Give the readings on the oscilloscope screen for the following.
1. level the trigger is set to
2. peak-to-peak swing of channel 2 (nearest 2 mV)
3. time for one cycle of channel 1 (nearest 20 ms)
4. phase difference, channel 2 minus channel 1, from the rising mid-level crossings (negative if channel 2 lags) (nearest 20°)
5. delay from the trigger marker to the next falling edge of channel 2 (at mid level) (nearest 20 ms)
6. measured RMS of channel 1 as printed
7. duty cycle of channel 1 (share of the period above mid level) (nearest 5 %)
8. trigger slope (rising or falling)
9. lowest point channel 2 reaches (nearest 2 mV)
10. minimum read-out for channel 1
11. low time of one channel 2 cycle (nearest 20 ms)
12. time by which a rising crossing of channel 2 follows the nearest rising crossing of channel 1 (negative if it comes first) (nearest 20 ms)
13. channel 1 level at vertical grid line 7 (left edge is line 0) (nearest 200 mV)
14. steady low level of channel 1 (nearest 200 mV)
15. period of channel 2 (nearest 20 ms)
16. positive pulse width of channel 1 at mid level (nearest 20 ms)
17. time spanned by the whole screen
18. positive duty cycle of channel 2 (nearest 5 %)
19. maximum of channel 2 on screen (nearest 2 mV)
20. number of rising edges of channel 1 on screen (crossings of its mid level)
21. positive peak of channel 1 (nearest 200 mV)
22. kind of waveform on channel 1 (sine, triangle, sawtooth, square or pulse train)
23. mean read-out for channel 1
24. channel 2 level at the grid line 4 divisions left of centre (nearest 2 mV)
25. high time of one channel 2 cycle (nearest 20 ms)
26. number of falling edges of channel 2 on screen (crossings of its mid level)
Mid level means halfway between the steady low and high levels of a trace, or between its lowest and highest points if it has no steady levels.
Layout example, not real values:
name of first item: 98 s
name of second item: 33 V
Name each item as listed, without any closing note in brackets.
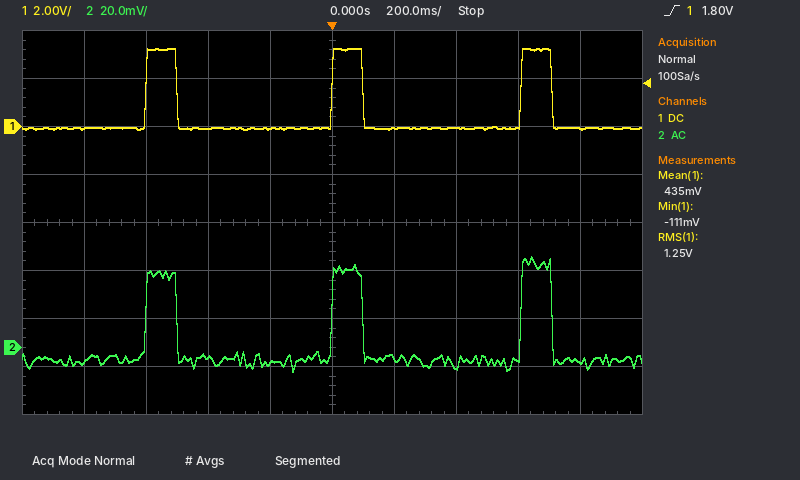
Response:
level the trigger is set to: 1.80 V
peak-to-peak swing of channel 2: 48 mV
time for one cycle of channel 1: 600 ms
phase difference, channel 2 minus channel 1, from the rising mid-level crossings (negative if channel 2 lags): 0°
delay from the trigger marker to the next falling edge of channel 2 (at mid level): 100 ms
measured RMS of channel 1 as printed: 1.25 V
duty cycle of channel 1 (share of the period above mid level): 15 %
trigger slope: rising
lowest point channel 2 reaches: -10 mV
minimum read-out for channel 1: -111 mV
low time of one channel 2 cycle: 500 ms
time by which a rising crossing of channel 2 follows the nearest rising crossing of channel 1 (negative if it comes first): 0 ms
channel 1 level at vertical grid line 7 (left edge is line 0): 0.0 V
steady low level of channel 1: 0.0 V
period of channel 2: 600 ms
positive pulse width of channel 1 at mid level: 100 ms
time spanned by the whole screen: 2 s
positive duty cycle of channel 2: 15 %
maximum of channel 2 on screen: 38 mV
number of rising edges of channel 1 on screen: 3
positive peak of channel 1: 3.2 V
kind of waveform on channel 1: pulse train
mean read-out for channel 1: 435 mV
channel 2 level at the grid line 4 divisions left of centre: -6 mV
high time of one channel 2 cycle: 100 ms
number of falling edges of channel 2 on screen: 3
